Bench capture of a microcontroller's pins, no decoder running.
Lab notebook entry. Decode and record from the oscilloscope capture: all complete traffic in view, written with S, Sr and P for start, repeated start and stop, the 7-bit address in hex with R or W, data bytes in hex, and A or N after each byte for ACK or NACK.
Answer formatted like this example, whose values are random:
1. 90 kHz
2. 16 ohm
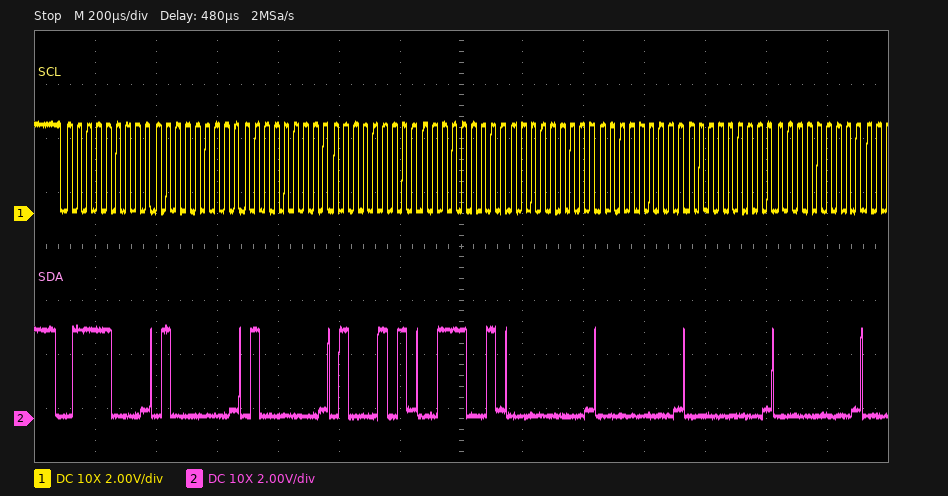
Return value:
1. S 3CW A 40 A 40 A 45 A 39 A 00 A 00 A 00 A 00 A
